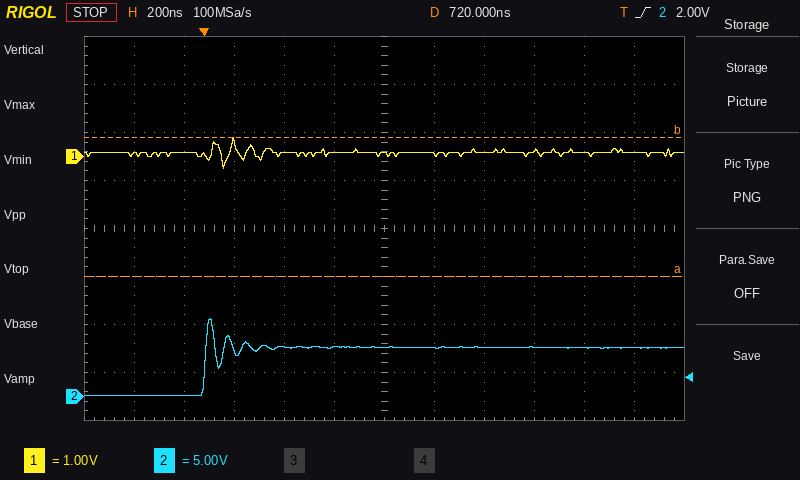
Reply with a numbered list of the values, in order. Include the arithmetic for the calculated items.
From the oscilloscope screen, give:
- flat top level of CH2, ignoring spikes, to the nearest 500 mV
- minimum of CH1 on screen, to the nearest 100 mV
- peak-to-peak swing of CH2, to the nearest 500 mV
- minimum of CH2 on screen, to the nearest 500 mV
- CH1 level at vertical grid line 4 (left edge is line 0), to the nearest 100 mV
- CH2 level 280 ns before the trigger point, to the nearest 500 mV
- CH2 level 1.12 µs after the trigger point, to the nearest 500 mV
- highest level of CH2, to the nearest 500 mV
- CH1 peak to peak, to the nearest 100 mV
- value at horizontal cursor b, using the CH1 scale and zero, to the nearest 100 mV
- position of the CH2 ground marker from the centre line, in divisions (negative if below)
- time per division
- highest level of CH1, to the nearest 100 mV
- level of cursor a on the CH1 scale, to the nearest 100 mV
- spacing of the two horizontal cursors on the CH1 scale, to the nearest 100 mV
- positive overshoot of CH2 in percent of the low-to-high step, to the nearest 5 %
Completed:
1. 5.0 V
2. -200 mV
3. 8.0 V − (0.0 V) = 8.0 V
4. 0.0 V
5. 100 mV
6. 0.0 V
7. 5.0 V
8. 8.0 V
9. 400 mV − (-200 mV) = 600 mV
10. 400 mV
11. -3.5 div
12. 200 ns
13. 400 mV
14. -2.5 V
15. 2.9 V
16. 60 %
